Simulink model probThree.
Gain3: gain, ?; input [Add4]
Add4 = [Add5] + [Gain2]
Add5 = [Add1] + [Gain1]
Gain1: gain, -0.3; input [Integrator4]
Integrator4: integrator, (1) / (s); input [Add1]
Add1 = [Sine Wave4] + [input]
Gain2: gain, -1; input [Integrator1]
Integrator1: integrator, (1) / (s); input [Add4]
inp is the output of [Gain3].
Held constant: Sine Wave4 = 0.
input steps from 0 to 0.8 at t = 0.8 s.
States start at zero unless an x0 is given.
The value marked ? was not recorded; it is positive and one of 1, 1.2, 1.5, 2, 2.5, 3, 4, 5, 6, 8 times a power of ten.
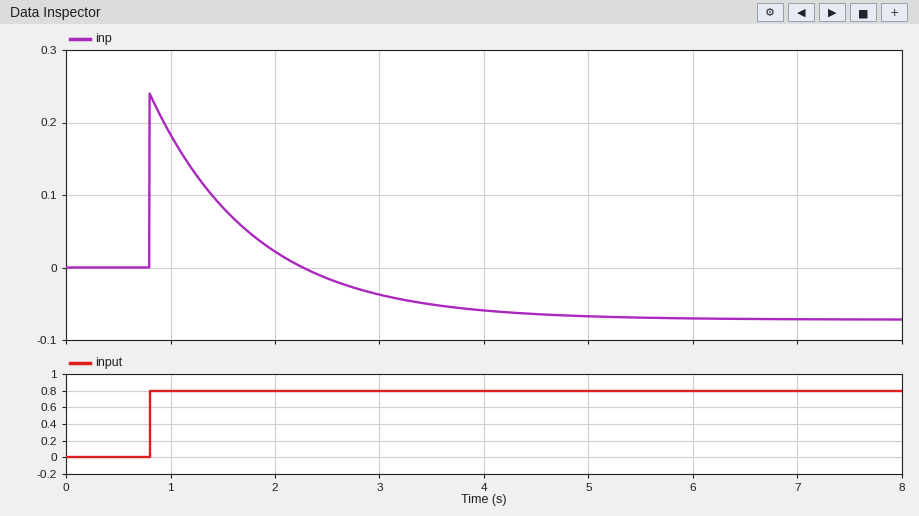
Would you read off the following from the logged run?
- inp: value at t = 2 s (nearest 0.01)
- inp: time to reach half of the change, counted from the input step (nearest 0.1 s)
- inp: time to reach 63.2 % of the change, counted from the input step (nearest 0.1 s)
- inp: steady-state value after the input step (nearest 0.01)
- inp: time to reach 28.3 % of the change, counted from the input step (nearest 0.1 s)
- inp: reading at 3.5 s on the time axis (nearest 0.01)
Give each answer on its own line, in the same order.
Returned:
0.02
2.2 s
2.5 s
-0.07
1.8 s
-0.05
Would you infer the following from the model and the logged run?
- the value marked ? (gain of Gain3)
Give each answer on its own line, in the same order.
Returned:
0.3
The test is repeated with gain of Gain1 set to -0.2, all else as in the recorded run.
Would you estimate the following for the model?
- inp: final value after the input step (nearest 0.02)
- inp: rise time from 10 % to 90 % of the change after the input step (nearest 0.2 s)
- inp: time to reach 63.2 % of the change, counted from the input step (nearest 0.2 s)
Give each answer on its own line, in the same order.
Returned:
-0.04
2.2 s
2.8 s
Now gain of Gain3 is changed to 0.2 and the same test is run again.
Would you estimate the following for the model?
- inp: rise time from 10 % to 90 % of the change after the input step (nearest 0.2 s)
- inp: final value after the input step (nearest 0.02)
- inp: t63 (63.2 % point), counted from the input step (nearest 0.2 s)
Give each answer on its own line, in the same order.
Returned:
2.2 s
-0.04
2.4 s
